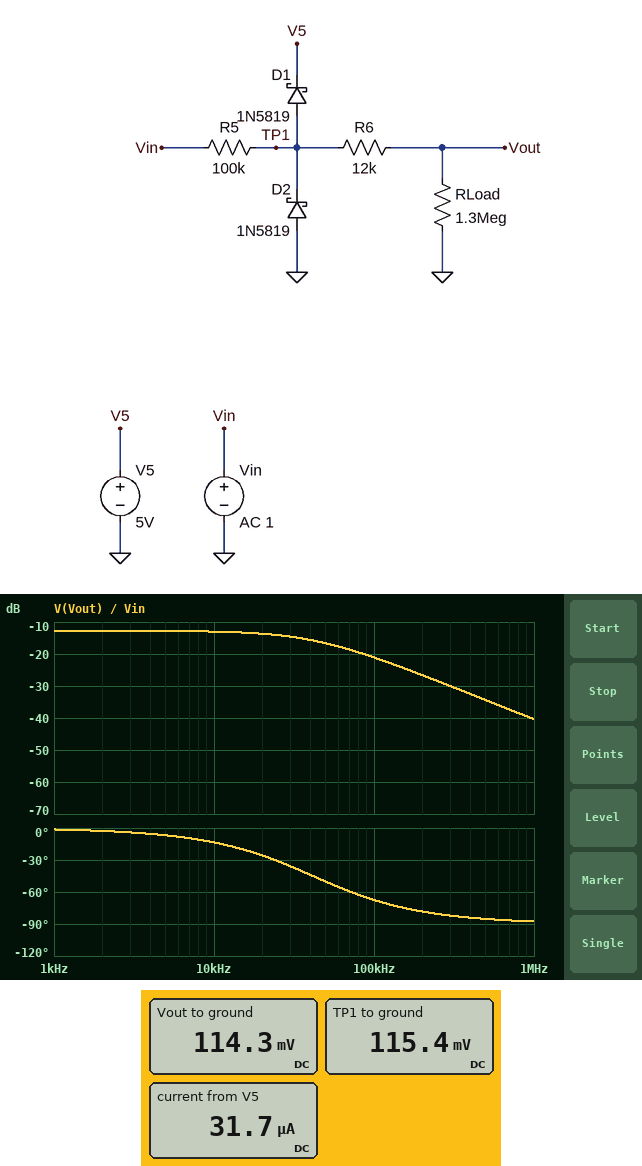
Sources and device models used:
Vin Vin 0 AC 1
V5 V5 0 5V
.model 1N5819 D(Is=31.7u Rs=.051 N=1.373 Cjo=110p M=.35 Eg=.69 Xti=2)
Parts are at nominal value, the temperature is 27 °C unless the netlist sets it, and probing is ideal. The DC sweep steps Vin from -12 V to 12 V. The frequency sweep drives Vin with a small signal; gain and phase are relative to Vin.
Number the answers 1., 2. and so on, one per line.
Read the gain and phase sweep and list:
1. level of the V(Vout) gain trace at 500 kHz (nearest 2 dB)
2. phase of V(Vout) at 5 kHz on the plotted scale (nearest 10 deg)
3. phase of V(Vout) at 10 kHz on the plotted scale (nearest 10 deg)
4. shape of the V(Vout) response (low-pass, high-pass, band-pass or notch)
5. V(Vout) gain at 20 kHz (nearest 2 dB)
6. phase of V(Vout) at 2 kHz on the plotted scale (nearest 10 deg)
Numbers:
1. -34 dB
2. -10 deg
3. -10 deg
4. low-pass
5. -14 dB
6. 0 deg
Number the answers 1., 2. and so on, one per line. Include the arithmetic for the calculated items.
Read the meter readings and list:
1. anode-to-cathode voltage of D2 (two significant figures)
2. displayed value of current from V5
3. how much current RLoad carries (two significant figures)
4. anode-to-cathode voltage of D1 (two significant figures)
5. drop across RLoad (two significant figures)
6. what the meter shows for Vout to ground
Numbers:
1. 0 V - 115.4 mV = -120 mV
2. 31.7 µA
3. (114.3 mV) / 1.3 MΩ = 88 nA
4. 115.4 mV - 5 V = -4.9 V
5. 114.3 mV = 110 mV
6. 114.3 mV
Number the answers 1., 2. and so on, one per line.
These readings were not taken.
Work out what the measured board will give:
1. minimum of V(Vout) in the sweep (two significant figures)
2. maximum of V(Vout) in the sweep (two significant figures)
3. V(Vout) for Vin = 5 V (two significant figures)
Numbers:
1. -47 mV
2. 5.0 V
3. 4.6 V
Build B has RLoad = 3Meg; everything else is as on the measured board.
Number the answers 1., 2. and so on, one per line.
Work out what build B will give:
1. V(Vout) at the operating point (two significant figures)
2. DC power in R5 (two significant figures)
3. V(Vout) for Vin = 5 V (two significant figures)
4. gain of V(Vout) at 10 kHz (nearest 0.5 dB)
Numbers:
1. 120 mV
2. 140 nW
3. 4.8 V
4. -12.5 dB
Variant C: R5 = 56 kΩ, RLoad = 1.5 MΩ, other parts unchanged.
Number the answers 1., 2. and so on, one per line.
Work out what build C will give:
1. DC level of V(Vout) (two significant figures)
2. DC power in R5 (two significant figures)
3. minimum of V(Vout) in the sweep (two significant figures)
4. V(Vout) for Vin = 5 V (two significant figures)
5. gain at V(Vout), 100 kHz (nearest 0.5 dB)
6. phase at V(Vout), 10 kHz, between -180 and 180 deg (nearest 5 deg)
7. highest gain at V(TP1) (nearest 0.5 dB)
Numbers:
1. 100 mV
2. 180 nW
3. -67 mV
4. 4.8 V
5. -17.0 dB
6. -10 deg
7. -12.0 dB
